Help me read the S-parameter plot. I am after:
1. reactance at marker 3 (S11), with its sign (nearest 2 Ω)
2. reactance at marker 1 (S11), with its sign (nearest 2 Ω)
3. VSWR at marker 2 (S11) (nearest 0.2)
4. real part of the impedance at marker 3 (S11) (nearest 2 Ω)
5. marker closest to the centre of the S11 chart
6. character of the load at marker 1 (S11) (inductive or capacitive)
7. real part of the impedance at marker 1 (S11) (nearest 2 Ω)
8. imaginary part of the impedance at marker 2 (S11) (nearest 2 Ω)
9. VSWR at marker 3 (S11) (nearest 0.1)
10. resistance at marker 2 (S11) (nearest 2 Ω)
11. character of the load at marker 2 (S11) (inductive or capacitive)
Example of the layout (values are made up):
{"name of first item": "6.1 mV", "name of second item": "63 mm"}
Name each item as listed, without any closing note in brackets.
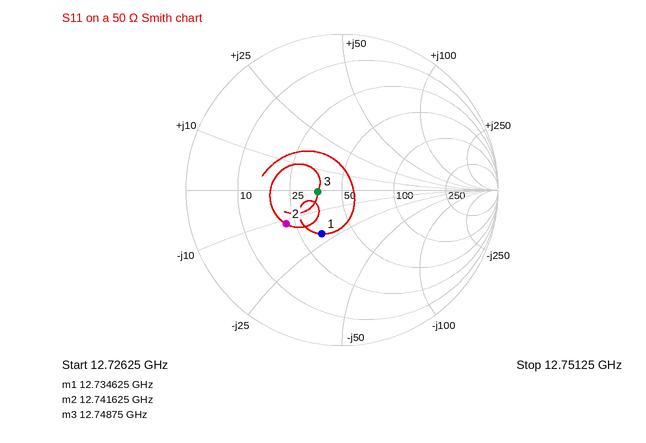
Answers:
{"reactance at marker 3 (S11), with its sign": "0 Ω", "reactance at marker 1 (S11), with its sign": "-20 Ω", "VSWR at marker 2 (S11)": "2.4", "real part of the impedance at marker 3 (S11)": "36 Ω", "marker closest to the centre of the S11 chart": "marker 3", "character of the load at marker 1 (S11)": "capacitive", "real part of the impedance at marker 1 (S11)": "34 Ω", "imaginary part of the impedance at marker 2 (S11)": "-12 Ω", "VSWR at marker 3 (S11)": "1.4", "resistance at marker 2 (S11)": "22 Ω", "character of the load at marker 2 (S11)": "capacitive"}
